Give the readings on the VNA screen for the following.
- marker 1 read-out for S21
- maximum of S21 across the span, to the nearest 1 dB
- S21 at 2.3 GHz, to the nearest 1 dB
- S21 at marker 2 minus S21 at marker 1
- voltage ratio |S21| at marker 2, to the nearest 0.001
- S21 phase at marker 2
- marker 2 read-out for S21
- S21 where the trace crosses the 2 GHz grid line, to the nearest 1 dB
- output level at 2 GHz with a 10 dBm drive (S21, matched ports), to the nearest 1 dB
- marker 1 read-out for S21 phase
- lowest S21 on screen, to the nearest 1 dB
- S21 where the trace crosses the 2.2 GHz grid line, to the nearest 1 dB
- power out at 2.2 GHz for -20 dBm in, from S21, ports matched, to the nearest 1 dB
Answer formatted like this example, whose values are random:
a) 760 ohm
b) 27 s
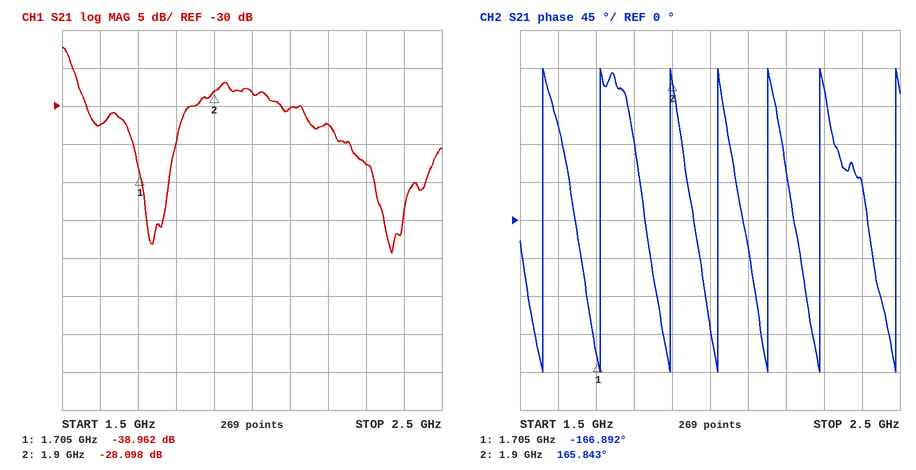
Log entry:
a) -38.962 dB
b) -22 dB
c) -38 dB
d) 10.864 dB
e) 0.039
f) 165.843°
g) -28.098 dB
h) -28 dB
i) -18 dBm
j) -166.892°
k) -49 dB
l) -32 dB
m) -52 dBm
